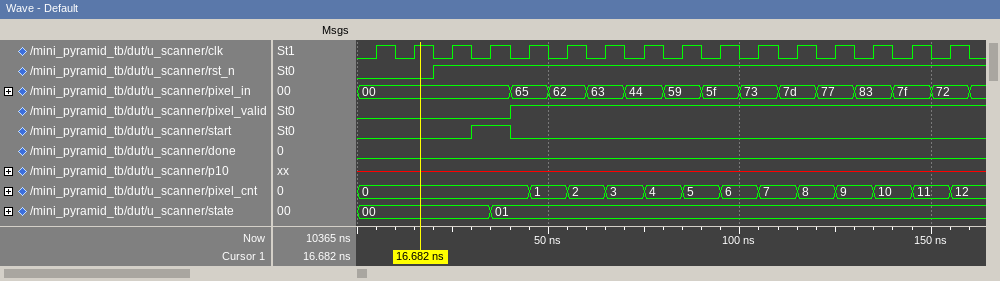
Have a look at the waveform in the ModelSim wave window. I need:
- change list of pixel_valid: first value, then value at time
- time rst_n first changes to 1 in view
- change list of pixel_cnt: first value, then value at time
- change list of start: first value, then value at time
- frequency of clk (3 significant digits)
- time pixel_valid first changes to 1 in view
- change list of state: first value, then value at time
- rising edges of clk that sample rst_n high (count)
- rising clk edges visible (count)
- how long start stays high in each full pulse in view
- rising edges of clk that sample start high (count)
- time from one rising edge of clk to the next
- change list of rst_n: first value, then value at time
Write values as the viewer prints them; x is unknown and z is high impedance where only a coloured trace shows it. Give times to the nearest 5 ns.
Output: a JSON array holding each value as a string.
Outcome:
["0, 1 at 40 ns", "20 ns", "0, 1 at 45 ns, 2 at 55 ns, 3 at 65 ns, 4 at 75 ns, 5 at 85 ns, 6 at 95 ns, 7 at 105 ns, 8 at 115 ns, 9 at 125 ns, 10 at 135 ns, 11 at 145 ns, 12 at 155 ns", "0, 1 at 30 ns, 0 at 40 ns", "100 MHz", "40 ns", "00, 01 at 35 ns", "14", "16", "10 ns", "1", "10 ns", "0, 1 at 20 ns"]
